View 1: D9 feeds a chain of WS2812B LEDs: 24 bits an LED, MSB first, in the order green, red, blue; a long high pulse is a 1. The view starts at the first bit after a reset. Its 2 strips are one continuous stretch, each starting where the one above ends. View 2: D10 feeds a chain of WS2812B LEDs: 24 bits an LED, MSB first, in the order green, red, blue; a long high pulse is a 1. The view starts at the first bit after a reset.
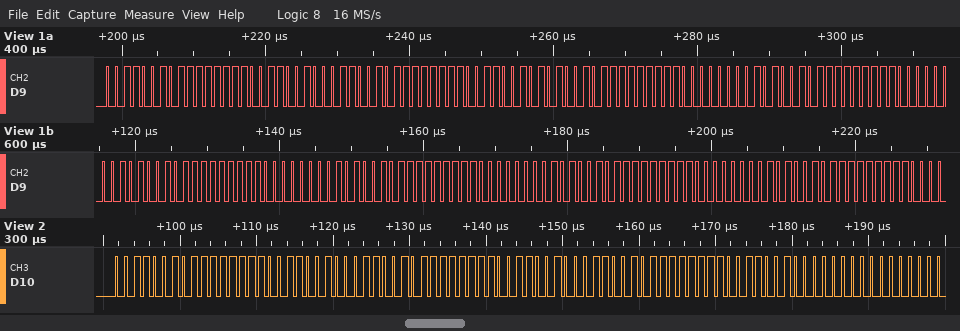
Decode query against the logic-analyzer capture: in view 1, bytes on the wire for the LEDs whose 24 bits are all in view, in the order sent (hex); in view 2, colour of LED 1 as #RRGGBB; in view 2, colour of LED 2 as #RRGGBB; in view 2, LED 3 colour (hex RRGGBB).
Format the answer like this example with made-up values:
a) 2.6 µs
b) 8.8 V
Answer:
a) 32 FF 32 32 FF 32 A5 FF 00 A5 FF 00 A5 FF 00 A5 FF 00 A5 FF 00
b) #FF3232
c) #FF3232
d) #FF3232
